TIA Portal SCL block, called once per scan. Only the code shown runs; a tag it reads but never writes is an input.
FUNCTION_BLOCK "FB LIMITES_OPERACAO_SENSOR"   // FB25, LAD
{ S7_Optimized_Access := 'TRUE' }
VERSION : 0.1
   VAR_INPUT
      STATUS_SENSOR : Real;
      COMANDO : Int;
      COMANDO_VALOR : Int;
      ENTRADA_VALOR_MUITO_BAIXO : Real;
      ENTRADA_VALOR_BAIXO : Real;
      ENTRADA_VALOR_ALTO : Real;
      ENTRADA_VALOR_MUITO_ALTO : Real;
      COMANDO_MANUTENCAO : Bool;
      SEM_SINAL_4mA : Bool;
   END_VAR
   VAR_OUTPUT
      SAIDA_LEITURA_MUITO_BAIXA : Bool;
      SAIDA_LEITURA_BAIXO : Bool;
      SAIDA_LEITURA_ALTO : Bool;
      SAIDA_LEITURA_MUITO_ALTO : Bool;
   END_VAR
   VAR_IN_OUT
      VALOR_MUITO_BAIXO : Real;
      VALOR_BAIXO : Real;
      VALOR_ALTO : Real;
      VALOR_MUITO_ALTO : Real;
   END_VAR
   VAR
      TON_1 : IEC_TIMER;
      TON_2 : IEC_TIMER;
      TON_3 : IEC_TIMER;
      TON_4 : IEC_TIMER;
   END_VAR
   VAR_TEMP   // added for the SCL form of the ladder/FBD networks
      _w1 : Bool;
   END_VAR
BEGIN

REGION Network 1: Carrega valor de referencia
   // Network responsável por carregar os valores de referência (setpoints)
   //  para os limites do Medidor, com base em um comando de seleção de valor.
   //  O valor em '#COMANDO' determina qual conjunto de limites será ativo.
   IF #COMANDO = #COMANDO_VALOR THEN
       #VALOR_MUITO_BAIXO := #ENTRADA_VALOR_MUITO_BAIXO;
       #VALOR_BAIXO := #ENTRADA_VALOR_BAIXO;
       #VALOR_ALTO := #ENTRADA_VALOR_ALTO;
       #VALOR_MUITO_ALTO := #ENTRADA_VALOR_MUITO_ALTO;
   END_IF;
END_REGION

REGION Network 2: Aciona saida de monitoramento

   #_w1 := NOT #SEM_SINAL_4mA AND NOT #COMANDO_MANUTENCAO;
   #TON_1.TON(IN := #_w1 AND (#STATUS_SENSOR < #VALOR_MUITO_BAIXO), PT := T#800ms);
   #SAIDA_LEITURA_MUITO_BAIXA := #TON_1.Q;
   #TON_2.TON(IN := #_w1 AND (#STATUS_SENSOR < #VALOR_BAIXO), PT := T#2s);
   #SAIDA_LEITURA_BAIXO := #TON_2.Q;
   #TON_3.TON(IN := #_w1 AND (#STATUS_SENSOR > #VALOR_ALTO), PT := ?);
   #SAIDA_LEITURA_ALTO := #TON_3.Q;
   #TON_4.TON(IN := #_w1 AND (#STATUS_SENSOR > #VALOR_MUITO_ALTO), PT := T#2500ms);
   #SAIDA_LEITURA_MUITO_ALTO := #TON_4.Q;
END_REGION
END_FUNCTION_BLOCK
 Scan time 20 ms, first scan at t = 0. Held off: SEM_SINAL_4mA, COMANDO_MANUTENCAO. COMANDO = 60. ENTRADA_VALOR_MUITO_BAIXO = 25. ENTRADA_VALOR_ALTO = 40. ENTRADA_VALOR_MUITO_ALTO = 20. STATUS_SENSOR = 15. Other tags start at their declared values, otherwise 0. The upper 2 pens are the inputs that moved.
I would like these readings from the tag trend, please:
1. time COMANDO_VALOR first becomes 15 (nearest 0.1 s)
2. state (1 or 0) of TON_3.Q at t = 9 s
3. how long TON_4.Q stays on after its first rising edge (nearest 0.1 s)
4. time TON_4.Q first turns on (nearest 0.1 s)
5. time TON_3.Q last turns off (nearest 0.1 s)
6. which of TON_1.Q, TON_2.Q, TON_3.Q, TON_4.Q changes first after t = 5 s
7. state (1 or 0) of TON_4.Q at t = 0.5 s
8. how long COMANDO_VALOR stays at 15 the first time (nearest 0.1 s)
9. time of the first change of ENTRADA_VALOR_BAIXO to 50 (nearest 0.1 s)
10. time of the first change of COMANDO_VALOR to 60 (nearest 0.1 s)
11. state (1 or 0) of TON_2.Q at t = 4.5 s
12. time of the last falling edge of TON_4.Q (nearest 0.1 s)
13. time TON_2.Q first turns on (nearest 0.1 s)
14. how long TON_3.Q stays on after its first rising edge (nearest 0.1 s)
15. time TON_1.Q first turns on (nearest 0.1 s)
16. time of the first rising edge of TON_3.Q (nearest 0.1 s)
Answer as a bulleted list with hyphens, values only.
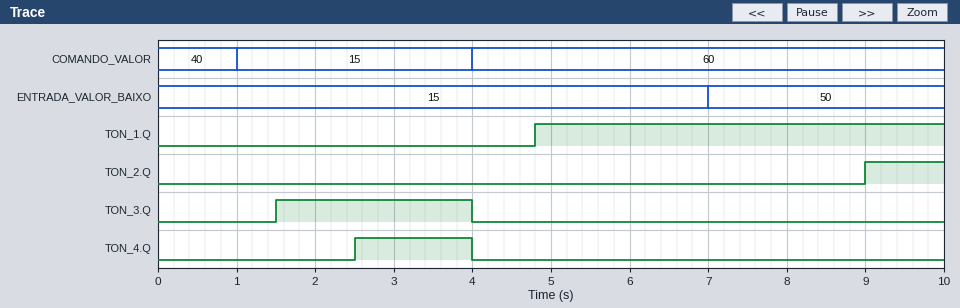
- 1.0 s
- 0
- 1.5 s
- 2.5 s
- 4.0 s
- TON_2.Q
- 0
- 3.0 s
- 7.0 s
- 4.0 s
- 0
- 4.0 s
- 9.0 s
- 2.5 s
- 4.8 s
- 1.5 s
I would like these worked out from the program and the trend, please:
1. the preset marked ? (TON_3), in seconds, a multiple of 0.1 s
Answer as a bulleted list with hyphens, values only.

- 1.5 s
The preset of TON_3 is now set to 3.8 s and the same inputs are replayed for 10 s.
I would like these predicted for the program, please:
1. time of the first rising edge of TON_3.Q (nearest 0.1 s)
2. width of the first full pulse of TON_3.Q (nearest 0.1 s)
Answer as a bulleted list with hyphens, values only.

- 3.8 s
- 0.2 s
